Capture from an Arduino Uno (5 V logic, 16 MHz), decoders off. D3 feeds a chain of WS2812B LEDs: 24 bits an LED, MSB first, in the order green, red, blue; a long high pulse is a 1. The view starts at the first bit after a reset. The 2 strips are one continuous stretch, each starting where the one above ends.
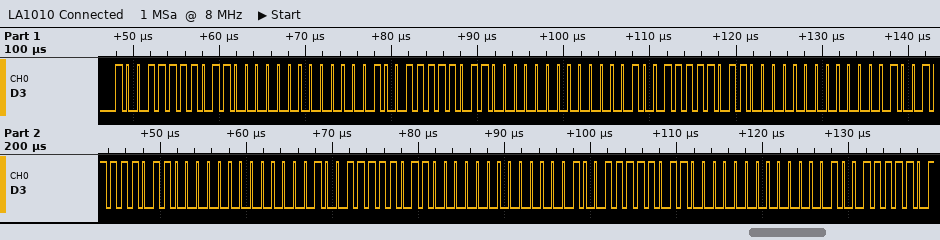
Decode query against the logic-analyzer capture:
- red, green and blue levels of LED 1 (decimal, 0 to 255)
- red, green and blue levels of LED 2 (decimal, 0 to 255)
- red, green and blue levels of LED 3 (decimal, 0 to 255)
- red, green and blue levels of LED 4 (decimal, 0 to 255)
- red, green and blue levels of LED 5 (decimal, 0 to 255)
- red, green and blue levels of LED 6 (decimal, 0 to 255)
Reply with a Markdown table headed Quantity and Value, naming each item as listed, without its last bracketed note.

| Quantity | Value |
|---|---|
| red, green and blue levels of LED 1 | 96, 159, 0 |
| red, green and blue levels of LED 2 | 96, 159, 0 |
| red, green and blue levels of LED 3 | 96, 159, 0 |
| red, green and blue levels of LED 4 | 96, 159, 0 |
| red, green and blue levels of LED 5 | 96, 159, 0 |
| red, green and blue levels of LED 6 | 96, 159, 0 |
